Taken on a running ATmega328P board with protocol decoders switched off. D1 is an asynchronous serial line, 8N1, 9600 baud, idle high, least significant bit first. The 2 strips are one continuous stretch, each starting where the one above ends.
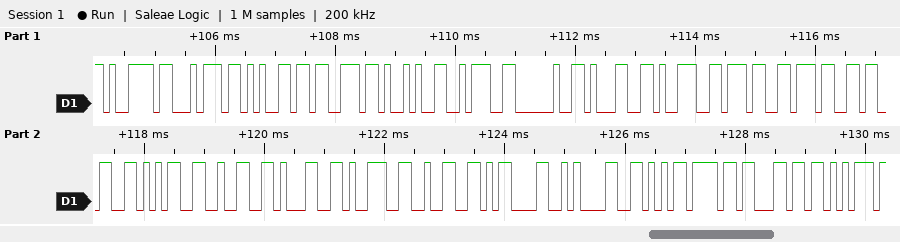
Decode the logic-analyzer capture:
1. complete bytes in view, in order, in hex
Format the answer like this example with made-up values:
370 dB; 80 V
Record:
0x79 0x74 0x65 0x73 0x29 0x3A 0x20 0x31 0x39 0x37 0x37 0x33 0x35 0x32 0x31 0x39 0x32 0x0D 0x0A 0x56 0x6F 0x6C 0x75
